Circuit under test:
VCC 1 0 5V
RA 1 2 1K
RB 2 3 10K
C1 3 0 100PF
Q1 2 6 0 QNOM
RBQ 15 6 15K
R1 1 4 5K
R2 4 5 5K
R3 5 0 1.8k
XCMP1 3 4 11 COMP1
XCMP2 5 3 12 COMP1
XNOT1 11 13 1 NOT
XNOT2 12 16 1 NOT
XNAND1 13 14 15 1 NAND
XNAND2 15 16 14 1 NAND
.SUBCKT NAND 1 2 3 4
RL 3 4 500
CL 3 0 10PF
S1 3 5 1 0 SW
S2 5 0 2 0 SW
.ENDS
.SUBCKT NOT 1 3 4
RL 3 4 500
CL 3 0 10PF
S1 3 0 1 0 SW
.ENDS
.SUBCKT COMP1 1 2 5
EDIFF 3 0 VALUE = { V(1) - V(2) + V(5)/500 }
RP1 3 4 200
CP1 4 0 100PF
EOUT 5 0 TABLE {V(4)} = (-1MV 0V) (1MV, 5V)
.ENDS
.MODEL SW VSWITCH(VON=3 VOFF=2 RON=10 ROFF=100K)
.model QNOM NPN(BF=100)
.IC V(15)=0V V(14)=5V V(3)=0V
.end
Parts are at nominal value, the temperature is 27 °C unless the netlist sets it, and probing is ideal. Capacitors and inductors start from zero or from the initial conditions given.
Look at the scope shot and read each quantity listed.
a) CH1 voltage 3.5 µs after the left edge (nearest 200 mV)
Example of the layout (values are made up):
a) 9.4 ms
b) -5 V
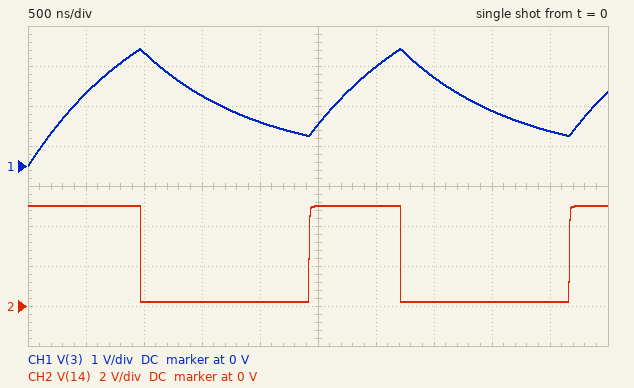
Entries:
a) 2.2 V
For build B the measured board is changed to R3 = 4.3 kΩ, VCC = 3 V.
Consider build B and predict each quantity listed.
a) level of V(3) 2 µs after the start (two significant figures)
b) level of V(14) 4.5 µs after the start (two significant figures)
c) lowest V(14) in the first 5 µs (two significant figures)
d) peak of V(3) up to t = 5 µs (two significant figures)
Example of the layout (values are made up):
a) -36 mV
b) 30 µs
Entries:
a) 920 mV
b) 3.0 V
c) 130 mV
d) 2.0 V
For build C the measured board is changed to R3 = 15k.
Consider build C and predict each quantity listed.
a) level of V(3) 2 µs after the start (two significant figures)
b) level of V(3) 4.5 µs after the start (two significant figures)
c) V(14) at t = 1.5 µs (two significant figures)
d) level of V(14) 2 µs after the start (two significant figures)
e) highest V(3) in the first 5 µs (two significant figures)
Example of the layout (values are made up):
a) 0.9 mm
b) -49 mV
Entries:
a) 3.3 V
b) 3.1 V
c) 5.0 V
d) 190 mV
e) 4.0 V
